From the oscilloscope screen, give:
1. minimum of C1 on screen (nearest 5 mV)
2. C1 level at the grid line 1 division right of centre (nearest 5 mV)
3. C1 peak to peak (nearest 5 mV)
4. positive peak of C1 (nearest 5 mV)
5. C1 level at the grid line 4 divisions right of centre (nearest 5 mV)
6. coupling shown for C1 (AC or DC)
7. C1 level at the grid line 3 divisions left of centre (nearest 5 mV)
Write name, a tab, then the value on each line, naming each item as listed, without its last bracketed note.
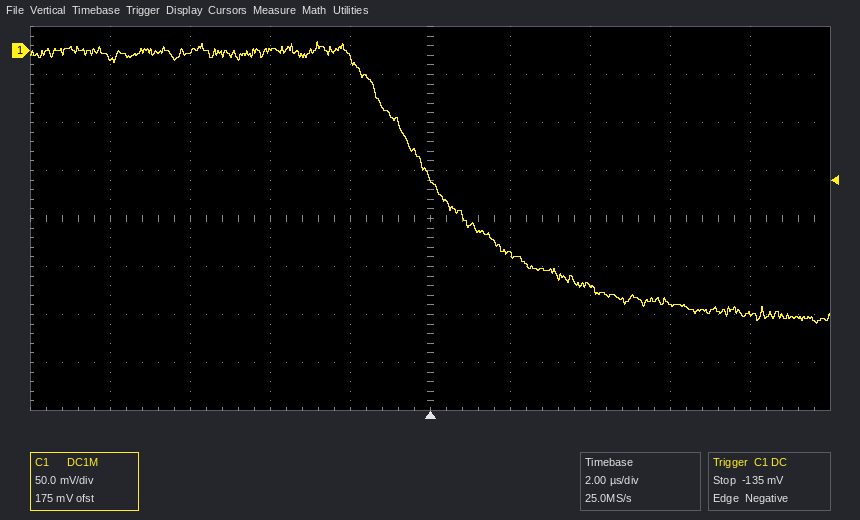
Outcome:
minimum of C1 on screen	-285 mV
C1 level at the grid line 1 division right of centre	-215 mV
C1 peak to peak	295 mV
positive peak of C1	10 mV
C1 level at the grid line 4 divisions right of centre	-275 mV
coupling shown for C1	DC
C1 level at the grid line 3 divisions left of centre	0 mV
